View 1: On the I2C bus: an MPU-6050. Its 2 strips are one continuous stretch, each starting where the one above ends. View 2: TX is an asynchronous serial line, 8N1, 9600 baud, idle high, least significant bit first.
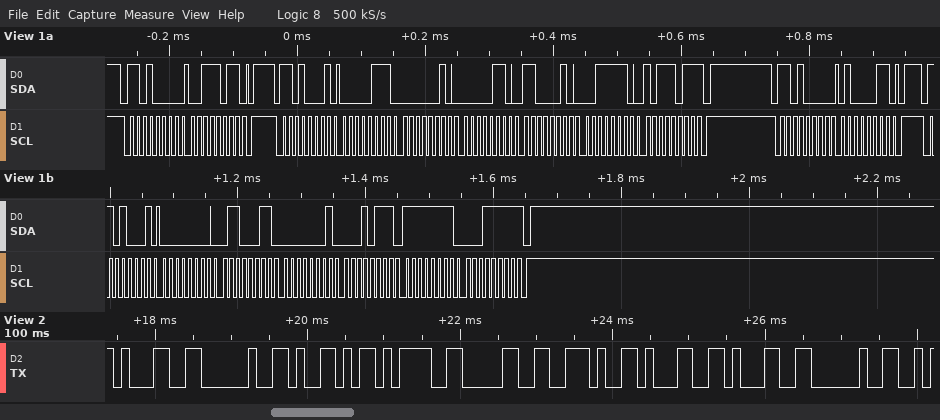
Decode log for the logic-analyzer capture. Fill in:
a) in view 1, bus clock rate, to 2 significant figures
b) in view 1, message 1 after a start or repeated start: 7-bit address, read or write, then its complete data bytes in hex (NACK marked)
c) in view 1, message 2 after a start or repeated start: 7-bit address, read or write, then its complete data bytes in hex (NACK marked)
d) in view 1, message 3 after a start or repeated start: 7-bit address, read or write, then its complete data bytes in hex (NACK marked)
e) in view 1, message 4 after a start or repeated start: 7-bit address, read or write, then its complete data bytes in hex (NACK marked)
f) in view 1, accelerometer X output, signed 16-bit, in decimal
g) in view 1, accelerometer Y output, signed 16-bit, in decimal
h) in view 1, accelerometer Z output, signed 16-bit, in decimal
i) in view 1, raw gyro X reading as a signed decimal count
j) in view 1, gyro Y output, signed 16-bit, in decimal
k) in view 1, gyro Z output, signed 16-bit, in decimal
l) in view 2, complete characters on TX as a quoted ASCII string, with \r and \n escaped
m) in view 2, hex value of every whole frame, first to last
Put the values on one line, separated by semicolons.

100 kHz; 0x68 write: 3B; 0x68 read: 07 02 06 C2 3E BB NACK; 0x68 write: 43; 0x68 read: 00 63 01 17 FF 1F NACK; 1794; 1730; 16059; 99; 279; -225; "1 Y=0.11 "; 31 20 59 3D 30 2E 31 31 20
